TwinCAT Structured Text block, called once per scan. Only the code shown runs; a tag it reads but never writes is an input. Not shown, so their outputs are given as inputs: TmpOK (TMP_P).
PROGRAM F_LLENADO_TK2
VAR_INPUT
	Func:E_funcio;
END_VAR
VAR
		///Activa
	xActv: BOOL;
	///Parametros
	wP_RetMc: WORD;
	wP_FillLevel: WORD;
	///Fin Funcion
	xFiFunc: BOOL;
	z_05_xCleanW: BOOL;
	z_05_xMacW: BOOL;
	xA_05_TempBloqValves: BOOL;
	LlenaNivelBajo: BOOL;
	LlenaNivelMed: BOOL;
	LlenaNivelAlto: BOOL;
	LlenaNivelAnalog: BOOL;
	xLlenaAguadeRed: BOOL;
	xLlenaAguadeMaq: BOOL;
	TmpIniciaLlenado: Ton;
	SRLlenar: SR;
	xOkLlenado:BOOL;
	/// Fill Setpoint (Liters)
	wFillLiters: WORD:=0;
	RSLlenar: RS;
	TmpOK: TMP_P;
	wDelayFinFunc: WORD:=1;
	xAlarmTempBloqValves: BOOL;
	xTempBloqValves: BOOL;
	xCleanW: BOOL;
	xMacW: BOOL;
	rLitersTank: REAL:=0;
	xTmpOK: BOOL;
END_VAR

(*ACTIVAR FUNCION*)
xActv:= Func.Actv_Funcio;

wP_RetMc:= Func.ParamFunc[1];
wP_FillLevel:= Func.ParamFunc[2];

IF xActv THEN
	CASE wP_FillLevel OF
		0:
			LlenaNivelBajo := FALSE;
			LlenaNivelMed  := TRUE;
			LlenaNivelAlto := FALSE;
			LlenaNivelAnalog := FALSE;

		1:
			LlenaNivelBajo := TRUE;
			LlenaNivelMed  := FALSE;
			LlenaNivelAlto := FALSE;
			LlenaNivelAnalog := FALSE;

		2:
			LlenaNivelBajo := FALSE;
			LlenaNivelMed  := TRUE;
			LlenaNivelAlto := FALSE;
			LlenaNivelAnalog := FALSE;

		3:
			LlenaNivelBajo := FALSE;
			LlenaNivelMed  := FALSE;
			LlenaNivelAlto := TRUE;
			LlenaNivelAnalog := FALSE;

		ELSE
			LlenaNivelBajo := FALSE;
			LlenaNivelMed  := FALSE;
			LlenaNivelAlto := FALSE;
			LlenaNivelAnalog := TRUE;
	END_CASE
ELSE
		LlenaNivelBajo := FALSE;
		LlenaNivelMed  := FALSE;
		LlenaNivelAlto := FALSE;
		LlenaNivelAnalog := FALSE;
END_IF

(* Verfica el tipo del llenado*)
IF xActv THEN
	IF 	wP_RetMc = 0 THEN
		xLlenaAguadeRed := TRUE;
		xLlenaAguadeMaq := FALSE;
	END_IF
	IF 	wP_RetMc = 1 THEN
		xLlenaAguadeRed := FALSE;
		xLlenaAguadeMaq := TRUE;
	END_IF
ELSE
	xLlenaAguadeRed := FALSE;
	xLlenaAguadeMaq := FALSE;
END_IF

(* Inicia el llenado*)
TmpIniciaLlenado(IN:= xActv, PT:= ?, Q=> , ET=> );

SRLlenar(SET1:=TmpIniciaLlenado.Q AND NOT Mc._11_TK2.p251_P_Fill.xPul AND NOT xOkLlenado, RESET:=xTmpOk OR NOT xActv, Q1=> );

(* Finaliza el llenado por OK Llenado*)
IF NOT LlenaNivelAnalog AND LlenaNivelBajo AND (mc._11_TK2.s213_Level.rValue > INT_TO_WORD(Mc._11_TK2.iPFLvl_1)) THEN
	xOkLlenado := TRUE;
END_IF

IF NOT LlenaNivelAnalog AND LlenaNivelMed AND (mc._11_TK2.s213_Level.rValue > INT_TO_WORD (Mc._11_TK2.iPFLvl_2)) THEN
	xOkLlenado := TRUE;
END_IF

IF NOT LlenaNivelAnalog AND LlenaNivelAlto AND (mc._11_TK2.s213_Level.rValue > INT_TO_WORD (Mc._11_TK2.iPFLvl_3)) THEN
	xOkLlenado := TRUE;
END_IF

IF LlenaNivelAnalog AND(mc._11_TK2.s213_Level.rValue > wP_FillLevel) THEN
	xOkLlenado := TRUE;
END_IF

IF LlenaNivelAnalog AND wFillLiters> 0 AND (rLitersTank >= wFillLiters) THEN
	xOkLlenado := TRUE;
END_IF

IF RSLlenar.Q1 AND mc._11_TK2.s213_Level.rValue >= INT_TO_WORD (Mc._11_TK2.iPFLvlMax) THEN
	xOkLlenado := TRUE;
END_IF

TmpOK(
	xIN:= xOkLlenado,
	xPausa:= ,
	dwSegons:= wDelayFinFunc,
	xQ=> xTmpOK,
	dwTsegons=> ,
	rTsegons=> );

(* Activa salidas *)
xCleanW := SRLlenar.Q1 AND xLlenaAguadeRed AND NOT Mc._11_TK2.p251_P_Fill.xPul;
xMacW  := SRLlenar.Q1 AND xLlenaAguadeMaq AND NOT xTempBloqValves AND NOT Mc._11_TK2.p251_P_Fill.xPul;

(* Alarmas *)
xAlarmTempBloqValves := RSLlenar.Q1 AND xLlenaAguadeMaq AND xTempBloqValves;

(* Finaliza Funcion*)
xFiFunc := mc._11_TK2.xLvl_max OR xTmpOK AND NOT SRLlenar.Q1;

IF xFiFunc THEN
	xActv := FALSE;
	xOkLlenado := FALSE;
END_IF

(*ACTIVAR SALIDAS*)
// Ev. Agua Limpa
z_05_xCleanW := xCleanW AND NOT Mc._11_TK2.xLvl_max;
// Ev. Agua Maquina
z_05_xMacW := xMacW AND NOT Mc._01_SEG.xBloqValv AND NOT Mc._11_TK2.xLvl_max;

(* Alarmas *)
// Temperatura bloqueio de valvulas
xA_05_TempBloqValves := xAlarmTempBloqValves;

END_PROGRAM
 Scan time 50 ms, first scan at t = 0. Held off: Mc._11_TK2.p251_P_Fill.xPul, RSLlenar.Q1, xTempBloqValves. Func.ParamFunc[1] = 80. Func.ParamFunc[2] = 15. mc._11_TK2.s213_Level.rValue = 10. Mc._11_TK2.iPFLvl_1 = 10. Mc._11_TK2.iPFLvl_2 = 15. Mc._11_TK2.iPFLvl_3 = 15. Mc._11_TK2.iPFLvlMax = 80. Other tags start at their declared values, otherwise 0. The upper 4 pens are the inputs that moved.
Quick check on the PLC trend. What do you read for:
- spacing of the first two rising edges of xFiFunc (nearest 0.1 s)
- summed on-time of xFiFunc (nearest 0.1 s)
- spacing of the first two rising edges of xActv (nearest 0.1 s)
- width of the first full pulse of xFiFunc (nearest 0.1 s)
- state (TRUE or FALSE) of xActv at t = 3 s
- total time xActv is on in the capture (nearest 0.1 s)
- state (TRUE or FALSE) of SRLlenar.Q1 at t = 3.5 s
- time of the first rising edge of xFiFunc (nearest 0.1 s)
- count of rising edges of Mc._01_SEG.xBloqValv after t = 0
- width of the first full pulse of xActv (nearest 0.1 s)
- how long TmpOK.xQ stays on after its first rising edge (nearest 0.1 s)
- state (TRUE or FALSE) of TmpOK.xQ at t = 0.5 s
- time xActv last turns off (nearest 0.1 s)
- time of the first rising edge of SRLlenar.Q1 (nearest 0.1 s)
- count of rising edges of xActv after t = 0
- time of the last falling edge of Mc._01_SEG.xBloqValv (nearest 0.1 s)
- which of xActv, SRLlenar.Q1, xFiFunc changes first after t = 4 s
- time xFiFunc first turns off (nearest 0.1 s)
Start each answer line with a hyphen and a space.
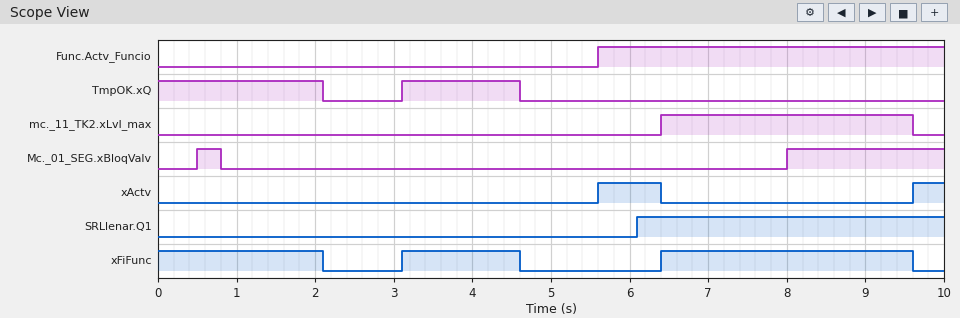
- 3.3 s
- 6.8 s
- 4.0 s
- 1.5 s
- FALSE
- 1.2 s
- FALSE
- 3.1 s
- 2
- 0.8 s
- 1.5 s
- TRUE
- 6.4 s
- 6.1 s
- 2
- 0.8 s
- xFiFunc
- 2.1 s
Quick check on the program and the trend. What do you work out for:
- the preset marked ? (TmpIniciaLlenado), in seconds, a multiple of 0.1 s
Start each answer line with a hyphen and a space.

- 0.5 s
